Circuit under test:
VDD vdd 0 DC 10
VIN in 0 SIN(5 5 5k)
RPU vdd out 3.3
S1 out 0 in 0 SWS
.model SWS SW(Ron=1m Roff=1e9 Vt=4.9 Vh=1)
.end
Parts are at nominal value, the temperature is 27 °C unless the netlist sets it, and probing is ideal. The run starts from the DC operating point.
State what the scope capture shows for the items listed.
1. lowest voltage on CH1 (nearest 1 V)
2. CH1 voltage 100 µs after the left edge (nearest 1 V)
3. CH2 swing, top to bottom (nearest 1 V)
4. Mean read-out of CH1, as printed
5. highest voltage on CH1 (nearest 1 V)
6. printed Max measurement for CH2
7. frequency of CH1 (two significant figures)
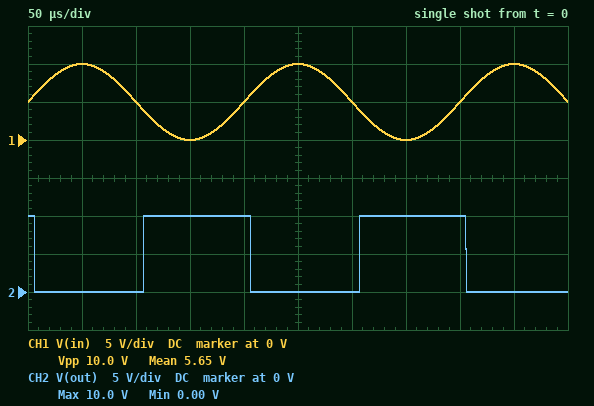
0 V
5 V
10 V
5.65 V
10 V
10.0 V
5.0 kHz
